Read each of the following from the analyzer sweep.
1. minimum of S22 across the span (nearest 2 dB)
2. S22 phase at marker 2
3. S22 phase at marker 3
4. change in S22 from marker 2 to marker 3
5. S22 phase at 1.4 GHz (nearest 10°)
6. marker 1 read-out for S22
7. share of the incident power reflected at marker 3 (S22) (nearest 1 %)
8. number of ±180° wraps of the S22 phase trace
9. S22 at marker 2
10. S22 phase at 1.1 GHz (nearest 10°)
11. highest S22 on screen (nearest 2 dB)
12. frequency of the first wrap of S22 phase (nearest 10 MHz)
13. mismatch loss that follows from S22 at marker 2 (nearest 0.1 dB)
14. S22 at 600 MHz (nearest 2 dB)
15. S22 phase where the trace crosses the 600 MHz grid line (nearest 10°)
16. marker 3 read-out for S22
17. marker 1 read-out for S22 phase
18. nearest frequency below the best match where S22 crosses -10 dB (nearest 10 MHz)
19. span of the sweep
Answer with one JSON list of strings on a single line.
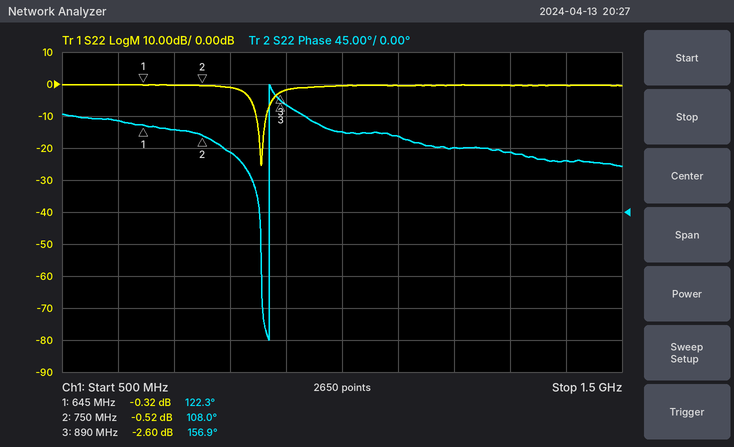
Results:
["-26 dB", "108.0°", "156.9°", "-2.08 dB", "70°", "-0.32 dB", "55 %", "1", "-0.52 dB", "110°", "0 dB", "870 MHz", "9.5 dB", "0 dB", "130°", "-2.60 dB", "122.3°", "850 MHz", "1 GHz"]
